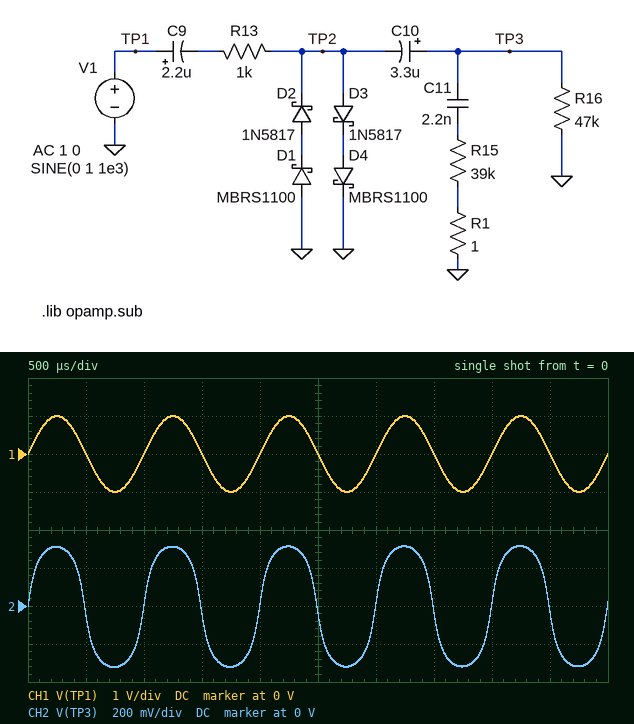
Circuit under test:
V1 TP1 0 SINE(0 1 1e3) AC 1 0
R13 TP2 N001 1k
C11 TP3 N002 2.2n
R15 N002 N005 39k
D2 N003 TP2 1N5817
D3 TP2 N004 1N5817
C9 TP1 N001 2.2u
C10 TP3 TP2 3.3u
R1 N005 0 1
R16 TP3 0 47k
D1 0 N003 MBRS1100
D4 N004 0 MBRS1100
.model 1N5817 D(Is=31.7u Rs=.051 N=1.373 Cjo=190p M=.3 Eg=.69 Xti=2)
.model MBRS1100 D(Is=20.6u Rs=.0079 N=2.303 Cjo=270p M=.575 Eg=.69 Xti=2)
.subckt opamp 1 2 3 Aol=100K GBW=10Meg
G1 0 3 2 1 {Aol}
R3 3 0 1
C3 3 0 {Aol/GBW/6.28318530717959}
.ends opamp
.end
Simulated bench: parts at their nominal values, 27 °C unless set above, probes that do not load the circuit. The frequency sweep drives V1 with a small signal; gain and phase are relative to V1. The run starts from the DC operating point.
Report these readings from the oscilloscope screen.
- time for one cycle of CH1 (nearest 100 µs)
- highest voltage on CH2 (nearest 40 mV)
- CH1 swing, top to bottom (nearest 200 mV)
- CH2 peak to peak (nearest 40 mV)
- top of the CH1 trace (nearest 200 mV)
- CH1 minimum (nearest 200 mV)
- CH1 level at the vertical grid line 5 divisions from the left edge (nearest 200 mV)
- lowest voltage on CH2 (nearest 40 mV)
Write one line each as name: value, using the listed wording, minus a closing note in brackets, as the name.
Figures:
time for one cycle of CH1: 1.0 ms
highest voltage on CH2: 320 mV
CH1 swing, top to bottom: 2.0 V
CH2 peak to peak: 640 mV
top of the CH1 trace: 1.0 V
CH1 minimum: -1.0 V
CH1 level at the vertical grid line 5 divisions from the left edge: 0 V
lowest voltage on CH2: -320 mV
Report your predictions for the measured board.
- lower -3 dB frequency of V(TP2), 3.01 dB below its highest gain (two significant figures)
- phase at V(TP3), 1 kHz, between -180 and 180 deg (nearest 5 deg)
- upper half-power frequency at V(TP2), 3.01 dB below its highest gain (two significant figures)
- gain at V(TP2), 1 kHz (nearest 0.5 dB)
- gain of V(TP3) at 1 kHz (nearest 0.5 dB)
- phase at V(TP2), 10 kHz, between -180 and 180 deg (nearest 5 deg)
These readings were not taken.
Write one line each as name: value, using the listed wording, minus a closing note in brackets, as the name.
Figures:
lower -3 dB frequency of V(TP2), 3.01 dB below its highest gain: 25 Hz
phase at V(TP3), 1 kHz, between -180 and 180 deg: 0 deg
upper half-power frequency at V(TP2), 3.01 dB below its highest gain: 850 kHz
gain at V(TP2), 1 kHz: -3.5 dB
gain of V(TP3) at 1 kHz: -3.5 dB
phase at V(TP2), 10 kHz, between -180 and 180 deg: 0 deg
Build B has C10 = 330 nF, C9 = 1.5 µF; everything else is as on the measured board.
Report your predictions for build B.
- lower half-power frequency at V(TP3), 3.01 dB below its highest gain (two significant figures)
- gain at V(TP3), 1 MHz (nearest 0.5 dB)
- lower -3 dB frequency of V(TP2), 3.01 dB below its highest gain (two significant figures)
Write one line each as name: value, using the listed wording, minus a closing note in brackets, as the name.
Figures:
lower half-power frequency at V(TP3), 3.01 dB below its highest gain: 39 Hz
gain at V(TP3), 1 MHz: -7.0 dB
lower -3 dB frequency of V(TP2), 3.01 dB below its highest gain: 36 Hz
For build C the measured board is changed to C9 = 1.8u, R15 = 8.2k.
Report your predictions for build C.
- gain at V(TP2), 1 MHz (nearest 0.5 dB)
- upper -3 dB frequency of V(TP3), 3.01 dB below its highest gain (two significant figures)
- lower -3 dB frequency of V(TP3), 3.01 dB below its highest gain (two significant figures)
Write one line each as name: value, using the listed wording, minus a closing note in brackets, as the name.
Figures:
gain at V(TP2), 1 MHz: -7.5 dB
upper -3 dB frequency of V(TP3), 3.01 dB below its highest gain: 750 kHz
lower -3 dB frequency of V(TP3), 3.01 dB below its highest gain: 30 Hz
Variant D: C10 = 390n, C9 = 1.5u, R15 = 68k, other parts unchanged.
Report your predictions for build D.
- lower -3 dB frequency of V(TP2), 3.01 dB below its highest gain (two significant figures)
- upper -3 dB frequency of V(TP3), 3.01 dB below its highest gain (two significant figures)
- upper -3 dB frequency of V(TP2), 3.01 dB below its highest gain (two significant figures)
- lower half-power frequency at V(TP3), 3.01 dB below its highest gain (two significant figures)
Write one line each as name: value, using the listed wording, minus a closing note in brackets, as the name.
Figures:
lower -3 dB frequency of V(TP2), 3.01 dB below its highest gain: 36 Hz
upper -3 dB frequency of V(TP3), 3.01 dB below its highest gain: 870 kHz
upper -3 dB frequency of V(TP2), 3.01 dB below its highest gain: 860 kHz
lower half-power frequency at V(TP3), 3.01 dB below its highest gain: 38 Hz
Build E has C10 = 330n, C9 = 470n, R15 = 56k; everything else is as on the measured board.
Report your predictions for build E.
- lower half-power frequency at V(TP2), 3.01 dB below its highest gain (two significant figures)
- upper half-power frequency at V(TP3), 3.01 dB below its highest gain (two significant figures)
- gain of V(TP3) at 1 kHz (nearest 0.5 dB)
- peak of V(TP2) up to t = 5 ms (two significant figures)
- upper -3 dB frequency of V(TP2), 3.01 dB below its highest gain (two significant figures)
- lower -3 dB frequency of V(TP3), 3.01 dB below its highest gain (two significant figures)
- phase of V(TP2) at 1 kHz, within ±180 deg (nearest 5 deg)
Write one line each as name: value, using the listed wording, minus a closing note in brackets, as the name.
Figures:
lower half-power frequency at V(TP2), 3.01 dB below its highest gain: 110 Hz
upper half-power frequency at V(TP3), 3.01 dB below its highest gain: 880 kHz
gain of V(TP3) at 1 kHz: -4.0 dB
peak of V(TP2) up to t = 5 ms: 310 mV
upper -3 dB frequency of V(TP2), 3.01 dB below its highest gain: 870 kHz
lower -3 dB frequency of V(TP3), 3.01 dB below its highest gain: 120 Hz
phase of V(TP2) at 1 kHz, within ±180 deg: 5 deg
